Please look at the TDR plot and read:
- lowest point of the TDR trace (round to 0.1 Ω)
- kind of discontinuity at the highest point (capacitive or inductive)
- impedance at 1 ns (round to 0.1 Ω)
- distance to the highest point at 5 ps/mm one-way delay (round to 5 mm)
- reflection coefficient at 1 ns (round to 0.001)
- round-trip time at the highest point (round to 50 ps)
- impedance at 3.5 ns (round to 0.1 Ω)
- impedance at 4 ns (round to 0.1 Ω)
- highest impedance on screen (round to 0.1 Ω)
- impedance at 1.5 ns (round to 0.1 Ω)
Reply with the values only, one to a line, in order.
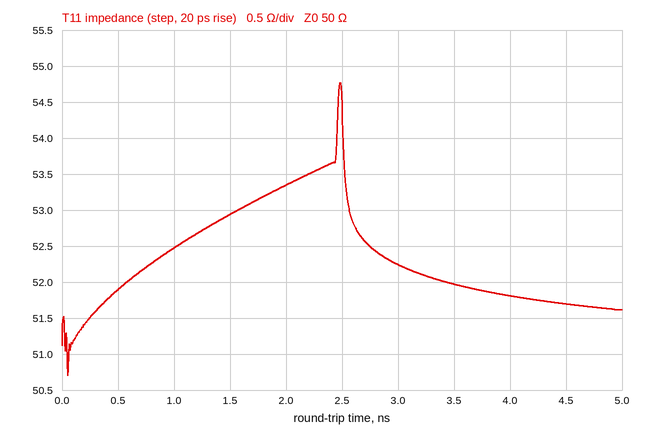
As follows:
50.7 Ω
inductive
52.5 Ω
250 mm
+0.024
2.50 ns
52.0 Ω
51.8 Ω
54.8 Ω
52.9 Ω
